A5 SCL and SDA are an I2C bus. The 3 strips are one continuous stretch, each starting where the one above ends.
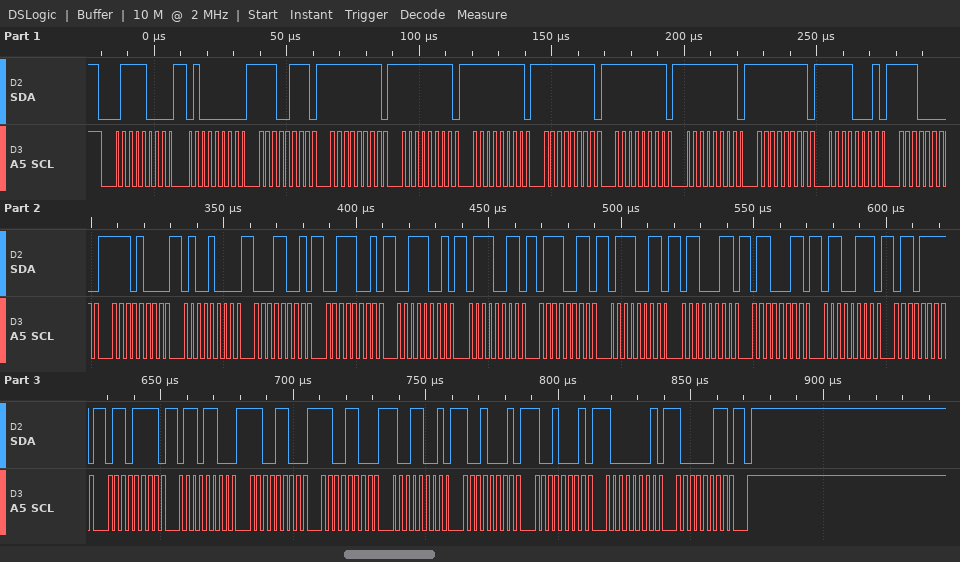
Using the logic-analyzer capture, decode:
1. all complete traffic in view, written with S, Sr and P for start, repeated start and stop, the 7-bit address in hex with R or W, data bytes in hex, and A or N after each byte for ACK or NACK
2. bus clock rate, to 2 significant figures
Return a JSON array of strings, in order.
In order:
["S 3CW A 40 A E7 A FF A FF A FF A FF A FF A FF A FF A F1 A E0 A E8 A 48 A 19 A 39 A 39 A 73 A 73 A 73 A 63 A 63 A 67 A 6F A 6F A 6C A CC A CC A 99 A 91 A 91 A 81 A 83 A P", "400 kHz"]
